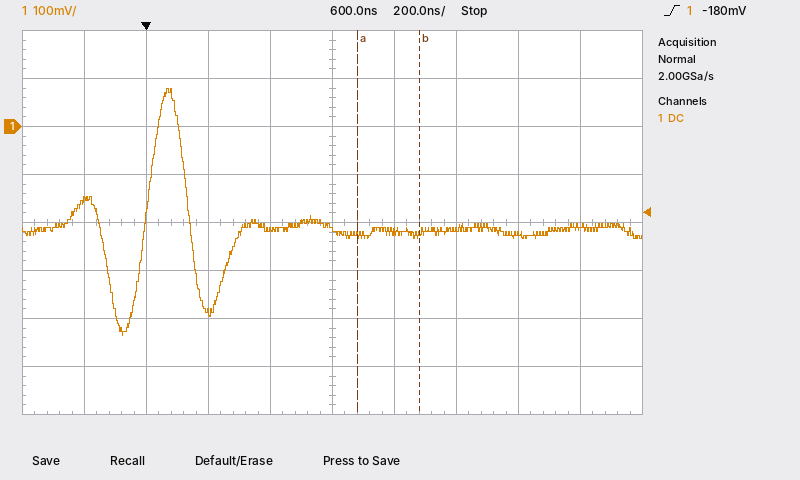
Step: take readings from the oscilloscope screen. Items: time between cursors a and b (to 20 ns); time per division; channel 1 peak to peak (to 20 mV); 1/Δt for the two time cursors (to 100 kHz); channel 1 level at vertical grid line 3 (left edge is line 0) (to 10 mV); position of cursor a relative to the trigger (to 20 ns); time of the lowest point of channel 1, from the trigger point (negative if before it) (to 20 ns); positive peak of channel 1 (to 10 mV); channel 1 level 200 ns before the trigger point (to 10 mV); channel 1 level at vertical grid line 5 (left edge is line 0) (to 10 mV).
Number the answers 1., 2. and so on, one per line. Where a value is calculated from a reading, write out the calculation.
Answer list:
1. 200 ns
2. 200 ns
3. 520 mV
4. 1 / 200 ns ≈ 5.0 MHz
5. -390 mV
6. +680 ns
7. -80 ns
8. 80 mV
9. -150 mV
10. -210 mV
